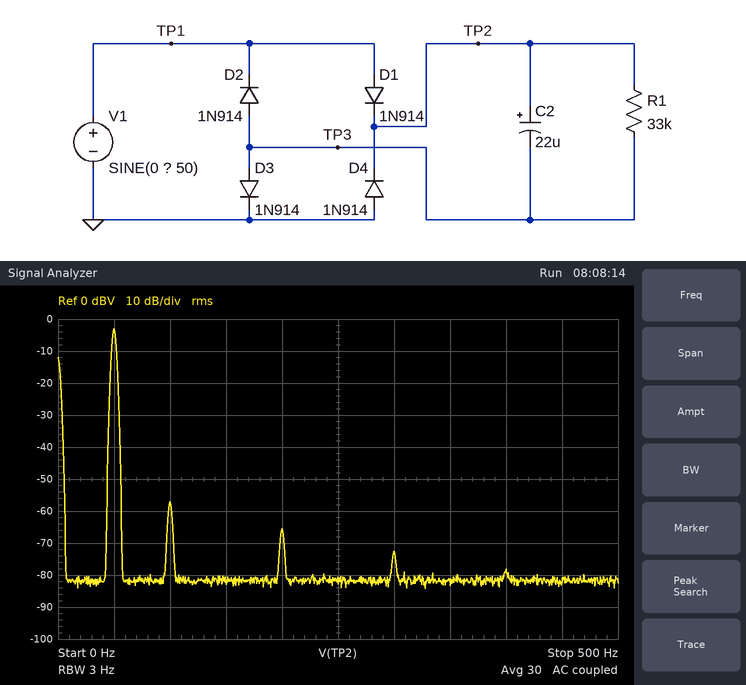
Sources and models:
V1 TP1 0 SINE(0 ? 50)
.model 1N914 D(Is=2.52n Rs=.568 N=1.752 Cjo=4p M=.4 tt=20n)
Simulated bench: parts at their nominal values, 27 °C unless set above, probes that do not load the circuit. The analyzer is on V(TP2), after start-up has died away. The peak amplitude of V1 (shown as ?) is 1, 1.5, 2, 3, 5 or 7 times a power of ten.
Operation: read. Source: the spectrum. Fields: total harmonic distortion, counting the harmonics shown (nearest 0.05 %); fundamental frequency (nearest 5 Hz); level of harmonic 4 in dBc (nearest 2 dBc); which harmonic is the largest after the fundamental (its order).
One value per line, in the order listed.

0.20 %
50 Hz
-62 dBc
2
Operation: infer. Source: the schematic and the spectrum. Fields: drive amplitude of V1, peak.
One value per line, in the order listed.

2 V
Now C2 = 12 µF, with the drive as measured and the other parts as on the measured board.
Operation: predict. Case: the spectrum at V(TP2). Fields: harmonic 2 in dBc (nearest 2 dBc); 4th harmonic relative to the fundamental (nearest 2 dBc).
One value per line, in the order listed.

-48 dBc
-58 dBc
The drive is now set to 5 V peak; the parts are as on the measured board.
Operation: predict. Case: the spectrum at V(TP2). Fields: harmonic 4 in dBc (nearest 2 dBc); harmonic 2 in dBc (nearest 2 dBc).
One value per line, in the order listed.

-56 dBc
-50 dBc
